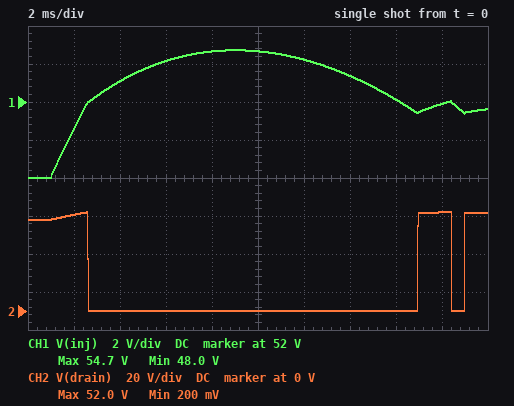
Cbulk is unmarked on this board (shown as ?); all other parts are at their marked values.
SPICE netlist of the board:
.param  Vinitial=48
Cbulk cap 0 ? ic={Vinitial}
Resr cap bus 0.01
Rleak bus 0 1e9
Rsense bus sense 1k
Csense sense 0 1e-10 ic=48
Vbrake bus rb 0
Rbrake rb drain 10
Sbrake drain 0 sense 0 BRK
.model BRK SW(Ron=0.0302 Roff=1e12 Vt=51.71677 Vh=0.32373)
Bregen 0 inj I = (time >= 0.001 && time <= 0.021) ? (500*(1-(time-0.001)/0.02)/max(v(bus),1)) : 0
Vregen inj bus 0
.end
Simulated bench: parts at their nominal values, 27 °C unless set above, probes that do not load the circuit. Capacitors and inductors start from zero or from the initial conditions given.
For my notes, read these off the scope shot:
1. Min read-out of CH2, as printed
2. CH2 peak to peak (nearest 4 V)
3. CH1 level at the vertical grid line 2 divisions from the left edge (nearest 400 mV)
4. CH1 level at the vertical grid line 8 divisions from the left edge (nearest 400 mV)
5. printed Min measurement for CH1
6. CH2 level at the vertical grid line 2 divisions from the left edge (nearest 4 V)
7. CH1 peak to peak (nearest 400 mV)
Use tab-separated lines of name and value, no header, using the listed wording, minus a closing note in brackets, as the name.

Min read-out of CH2, as printed	200 mV
CH2 peak to peak	52 V
CH1 level at the vertical grid line 2 divisions from the left edge	53.2 V
CH1 level at the vertical grid line 8 divisions from the left edge	52.0 V
printed Min measurement for CH1	48.0 V
CH2 level at the vertical grid line 2 divisions from the left edge	0 V
CH1 peak to peak	6.8 V
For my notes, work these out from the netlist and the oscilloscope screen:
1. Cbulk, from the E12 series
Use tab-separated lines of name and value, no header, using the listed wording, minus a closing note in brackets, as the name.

Cbulk, from the E12 series	3.9 mF
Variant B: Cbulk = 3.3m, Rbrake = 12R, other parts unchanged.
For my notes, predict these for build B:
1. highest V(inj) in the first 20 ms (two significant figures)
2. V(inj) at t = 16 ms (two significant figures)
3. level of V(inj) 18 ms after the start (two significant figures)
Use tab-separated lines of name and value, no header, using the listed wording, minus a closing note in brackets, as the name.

highest V(inj) in the first 20 ms	57 V
V(inj) at t = 16 ms	55 V
level of V(inj) 18 ms after the start	53 V
